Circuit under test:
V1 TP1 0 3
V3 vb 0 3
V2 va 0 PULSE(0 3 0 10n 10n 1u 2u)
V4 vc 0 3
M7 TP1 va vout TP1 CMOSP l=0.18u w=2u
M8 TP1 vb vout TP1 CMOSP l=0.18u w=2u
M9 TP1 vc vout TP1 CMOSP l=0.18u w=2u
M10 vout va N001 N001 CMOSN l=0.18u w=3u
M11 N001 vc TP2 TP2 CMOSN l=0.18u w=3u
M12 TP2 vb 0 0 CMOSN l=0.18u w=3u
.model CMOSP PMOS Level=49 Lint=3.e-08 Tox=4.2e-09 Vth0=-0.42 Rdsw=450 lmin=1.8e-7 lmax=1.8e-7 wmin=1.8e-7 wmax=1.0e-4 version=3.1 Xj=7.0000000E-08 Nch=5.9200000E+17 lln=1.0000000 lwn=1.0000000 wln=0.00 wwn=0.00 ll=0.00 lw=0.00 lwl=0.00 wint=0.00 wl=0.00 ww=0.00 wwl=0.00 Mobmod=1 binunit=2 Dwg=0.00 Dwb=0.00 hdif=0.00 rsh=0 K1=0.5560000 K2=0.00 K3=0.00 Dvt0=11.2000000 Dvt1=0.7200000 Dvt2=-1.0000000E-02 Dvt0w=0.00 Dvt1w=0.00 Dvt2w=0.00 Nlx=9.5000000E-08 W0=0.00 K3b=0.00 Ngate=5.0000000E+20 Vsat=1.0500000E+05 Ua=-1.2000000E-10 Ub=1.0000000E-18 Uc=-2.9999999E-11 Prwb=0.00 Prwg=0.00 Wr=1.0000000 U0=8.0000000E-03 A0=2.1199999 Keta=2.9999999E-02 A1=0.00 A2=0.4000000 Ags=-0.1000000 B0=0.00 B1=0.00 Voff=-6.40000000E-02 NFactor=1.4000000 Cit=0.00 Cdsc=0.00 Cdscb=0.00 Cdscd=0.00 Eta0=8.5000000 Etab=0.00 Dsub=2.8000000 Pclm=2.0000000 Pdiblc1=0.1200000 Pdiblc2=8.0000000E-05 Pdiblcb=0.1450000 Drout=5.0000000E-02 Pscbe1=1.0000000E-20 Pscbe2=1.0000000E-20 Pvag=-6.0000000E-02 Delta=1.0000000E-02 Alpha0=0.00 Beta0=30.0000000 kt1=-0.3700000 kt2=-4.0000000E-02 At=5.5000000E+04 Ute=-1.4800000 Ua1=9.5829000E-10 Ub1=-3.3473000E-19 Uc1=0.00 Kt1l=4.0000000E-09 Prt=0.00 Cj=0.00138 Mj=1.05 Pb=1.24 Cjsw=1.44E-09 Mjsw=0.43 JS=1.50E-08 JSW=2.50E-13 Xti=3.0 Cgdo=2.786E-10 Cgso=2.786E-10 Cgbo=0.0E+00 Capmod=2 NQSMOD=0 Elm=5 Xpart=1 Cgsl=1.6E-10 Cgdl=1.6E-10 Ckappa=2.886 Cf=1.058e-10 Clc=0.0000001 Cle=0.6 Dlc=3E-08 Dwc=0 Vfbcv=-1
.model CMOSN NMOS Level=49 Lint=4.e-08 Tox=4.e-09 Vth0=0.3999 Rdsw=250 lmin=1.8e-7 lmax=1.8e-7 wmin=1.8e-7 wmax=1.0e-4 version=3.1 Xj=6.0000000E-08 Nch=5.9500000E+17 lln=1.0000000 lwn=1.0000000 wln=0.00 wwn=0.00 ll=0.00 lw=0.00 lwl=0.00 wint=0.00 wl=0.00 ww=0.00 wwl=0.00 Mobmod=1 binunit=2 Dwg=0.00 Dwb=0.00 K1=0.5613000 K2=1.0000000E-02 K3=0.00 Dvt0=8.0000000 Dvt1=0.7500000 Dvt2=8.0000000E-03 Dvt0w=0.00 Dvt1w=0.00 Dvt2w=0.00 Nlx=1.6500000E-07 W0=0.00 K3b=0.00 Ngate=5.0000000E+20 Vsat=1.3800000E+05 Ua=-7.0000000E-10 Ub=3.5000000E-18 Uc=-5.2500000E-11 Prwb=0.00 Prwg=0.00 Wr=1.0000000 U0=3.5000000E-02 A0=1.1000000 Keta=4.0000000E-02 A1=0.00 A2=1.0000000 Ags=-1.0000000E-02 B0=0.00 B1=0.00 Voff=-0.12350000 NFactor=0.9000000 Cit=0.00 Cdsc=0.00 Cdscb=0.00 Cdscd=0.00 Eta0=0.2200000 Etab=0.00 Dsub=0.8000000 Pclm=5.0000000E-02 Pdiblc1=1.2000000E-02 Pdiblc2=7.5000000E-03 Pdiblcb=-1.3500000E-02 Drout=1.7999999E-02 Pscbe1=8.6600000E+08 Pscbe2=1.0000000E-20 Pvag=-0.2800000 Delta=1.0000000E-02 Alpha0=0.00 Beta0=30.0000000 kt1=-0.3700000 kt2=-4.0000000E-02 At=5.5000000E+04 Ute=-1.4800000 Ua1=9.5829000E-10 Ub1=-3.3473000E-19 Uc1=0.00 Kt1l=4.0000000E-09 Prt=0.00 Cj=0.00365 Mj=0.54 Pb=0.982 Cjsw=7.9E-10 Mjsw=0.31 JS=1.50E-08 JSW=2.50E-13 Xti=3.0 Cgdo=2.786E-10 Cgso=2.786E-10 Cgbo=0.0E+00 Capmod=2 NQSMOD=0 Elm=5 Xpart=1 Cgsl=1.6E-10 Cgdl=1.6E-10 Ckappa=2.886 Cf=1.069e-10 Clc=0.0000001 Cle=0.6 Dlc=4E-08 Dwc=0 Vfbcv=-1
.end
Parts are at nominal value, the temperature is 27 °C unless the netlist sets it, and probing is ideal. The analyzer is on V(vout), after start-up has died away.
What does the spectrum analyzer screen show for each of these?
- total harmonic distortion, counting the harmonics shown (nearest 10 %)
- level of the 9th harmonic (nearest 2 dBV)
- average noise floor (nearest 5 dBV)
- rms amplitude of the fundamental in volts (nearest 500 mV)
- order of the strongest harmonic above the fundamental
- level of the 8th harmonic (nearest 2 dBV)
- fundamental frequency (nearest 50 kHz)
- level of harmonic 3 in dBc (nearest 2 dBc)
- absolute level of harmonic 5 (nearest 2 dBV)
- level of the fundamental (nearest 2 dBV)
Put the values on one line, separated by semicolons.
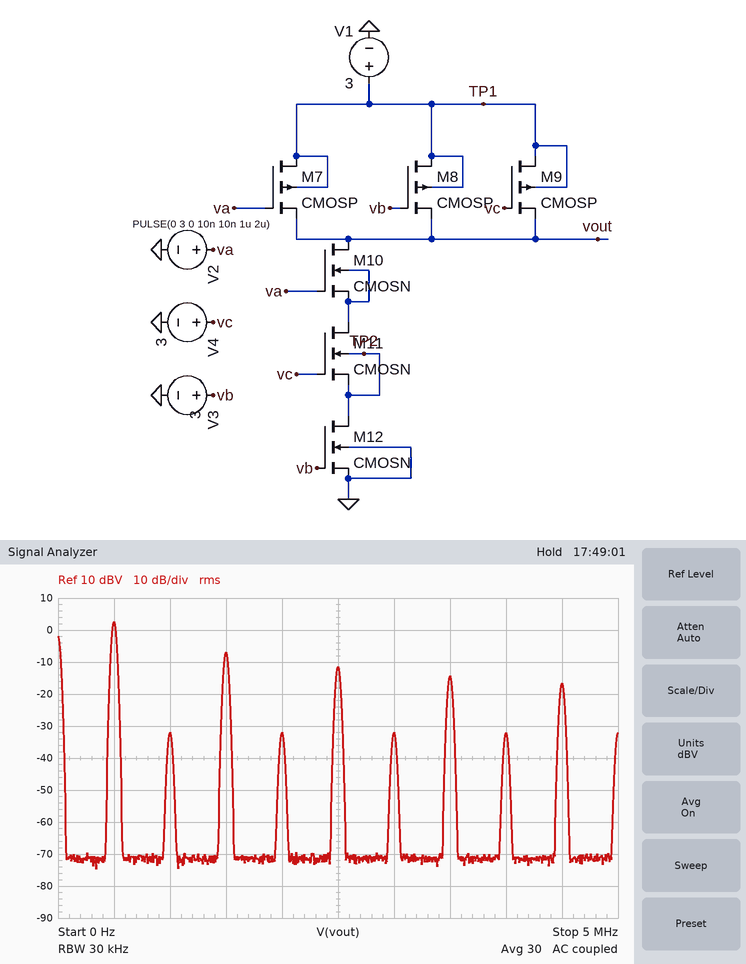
40 %; -16 dBV; -70 dBV; 1.5 V; 3; -32 dBV; 500 kHz; -10 dBc; -12 dBV; 2 dBV
